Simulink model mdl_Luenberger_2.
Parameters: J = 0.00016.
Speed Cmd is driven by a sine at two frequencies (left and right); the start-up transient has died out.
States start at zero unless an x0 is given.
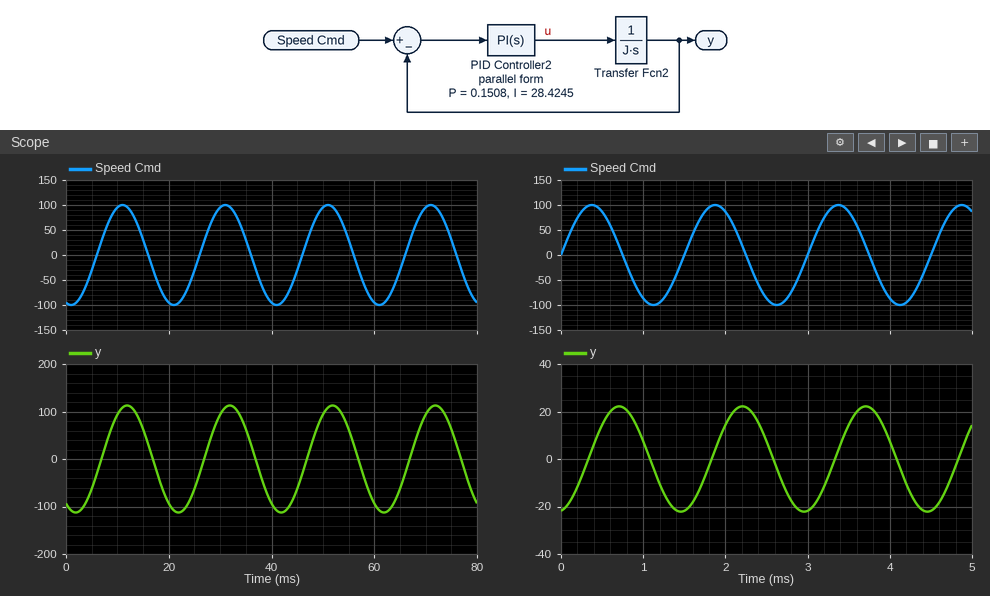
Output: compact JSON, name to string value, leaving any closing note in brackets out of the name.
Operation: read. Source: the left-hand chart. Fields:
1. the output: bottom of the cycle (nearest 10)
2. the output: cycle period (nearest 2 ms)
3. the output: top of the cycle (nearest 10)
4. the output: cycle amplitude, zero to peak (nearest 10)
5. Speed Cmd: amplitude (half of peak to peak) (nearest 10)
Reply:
{"the output: bottom of the cycle": "-110", "the output: cycle period": "20 ms", "the output: top of the cycle": "110", "the output: cycle amplitude, zero to peak": "110", "Speed Cmd: amplitude (half of peak to peak)": "100"}
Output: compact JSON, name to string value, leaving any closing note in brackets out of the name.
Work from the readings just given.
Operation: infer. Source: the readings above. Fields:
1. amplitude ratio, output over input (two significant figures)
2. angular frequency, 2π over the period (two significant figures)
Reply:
{"amplitude ratio, output over input": "1.1", "angular frequency, 2π over the period": "0.31 rad/ms"}
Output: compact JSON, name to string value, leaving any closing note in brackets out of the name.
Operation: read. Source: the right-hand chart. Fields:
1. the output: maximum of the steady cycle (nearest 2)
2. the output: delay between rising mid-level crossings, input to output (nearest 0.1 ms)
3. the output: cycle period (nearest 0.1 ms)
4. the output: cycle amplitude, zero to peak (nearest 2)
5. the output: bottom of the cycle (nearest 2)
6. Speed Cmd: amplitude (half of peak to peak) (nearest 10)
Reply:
{"the output: maximum of the steady cycle": "22", "the output: delay between rising mid-level crossings, input to output": "0.3 ms", "the output: cycle period": "1.5 ms", "the output: cycle amplitude, zero to peak": "22", "the output: bottom of the cycle": "-22", "Speed Cmd: amplitude (half of peak to peak)": "100"}
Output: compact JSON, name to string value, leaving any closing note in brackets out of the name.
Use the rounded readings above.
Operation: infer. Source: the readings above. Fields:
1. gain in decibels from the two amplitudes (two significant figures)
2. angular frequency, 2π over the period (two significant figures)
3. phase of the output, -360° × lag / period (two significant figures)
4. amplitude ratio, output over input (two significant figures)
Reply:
{"gain in decibels from the two amplitudes": "-13 dB", "angular frequency, 2π over the period": "4.2 rad/ms", "phase of the output, -360° × lag / period": "-72°", "amplitude ratio, output over input": "0.22"}
